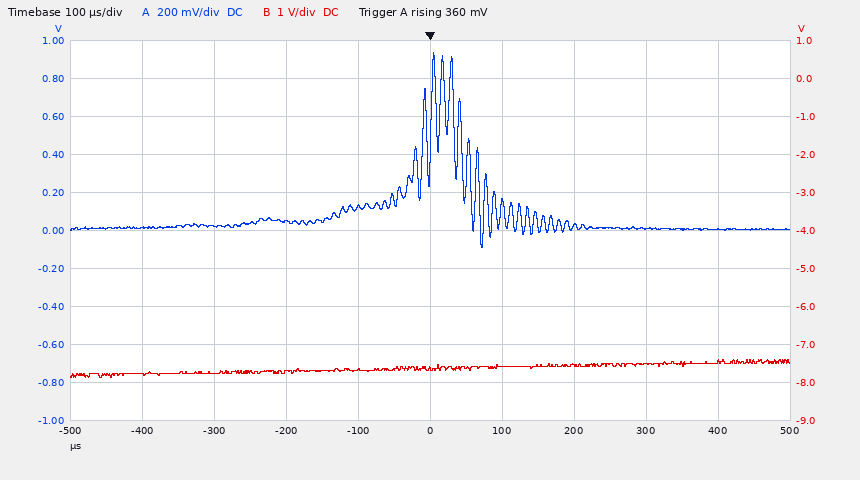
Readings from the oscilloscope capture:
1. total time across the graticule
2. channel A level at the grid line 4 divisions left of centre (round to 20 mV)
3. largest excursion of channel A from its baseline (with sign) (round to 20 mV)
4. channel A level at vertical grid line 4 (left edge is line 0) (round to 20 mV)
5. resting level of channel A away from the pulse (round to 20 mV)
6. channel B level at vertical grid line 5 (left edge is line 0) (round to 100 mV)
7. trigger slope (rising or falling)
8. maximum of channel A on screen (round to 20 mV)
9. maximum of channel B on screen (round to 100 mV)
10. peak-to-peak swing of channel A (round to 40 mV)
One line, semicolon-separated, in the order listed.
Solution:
1 ms; 20 mV; +920 mV; 120 mV; 20 mV; -7.6 V; rising; 940 mV; -7.4 V; 1.04 V
